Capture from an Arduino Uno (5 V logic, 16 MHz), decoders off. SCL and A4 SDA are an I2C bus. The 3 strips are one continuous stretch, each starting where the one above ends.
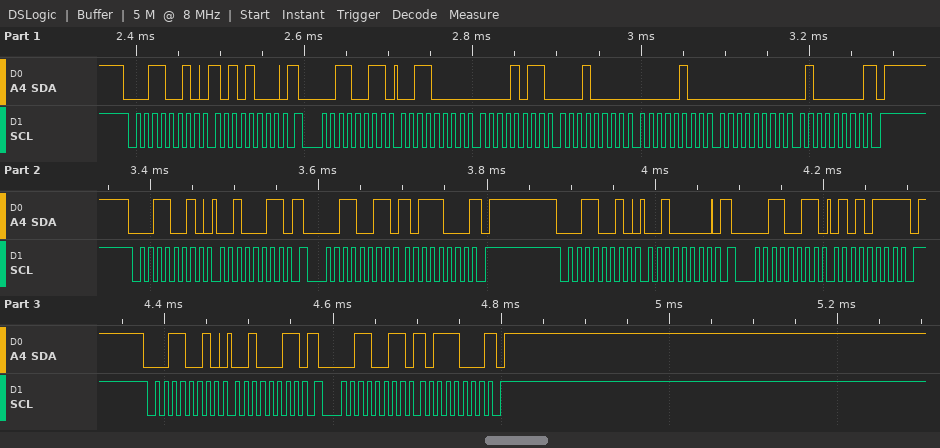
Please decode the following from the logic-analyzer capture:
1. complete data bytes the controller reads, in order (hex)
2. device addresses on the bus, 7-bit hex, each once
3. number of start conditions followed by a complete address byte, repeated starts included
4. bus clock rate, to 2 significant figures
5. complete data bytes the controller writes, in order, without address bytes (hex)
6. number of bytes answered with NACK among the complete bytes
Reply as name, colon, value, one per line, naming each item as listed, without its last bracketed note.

complete data bytes the controller reads, in order: 30 0B 10 04 00 40 B8 57 B8
device addresses on the bus, 7-bit hex, each once: 0x19
number of start conditions followed by a complete address byte, repeated starts included: 8
bus clock rate, to 2 significant figures: 100 kHz
complete data bytes the controller writes, in order, without address bytes: A8 23 20 23
number of bytes answered with NACK among the complete bytes: 4
